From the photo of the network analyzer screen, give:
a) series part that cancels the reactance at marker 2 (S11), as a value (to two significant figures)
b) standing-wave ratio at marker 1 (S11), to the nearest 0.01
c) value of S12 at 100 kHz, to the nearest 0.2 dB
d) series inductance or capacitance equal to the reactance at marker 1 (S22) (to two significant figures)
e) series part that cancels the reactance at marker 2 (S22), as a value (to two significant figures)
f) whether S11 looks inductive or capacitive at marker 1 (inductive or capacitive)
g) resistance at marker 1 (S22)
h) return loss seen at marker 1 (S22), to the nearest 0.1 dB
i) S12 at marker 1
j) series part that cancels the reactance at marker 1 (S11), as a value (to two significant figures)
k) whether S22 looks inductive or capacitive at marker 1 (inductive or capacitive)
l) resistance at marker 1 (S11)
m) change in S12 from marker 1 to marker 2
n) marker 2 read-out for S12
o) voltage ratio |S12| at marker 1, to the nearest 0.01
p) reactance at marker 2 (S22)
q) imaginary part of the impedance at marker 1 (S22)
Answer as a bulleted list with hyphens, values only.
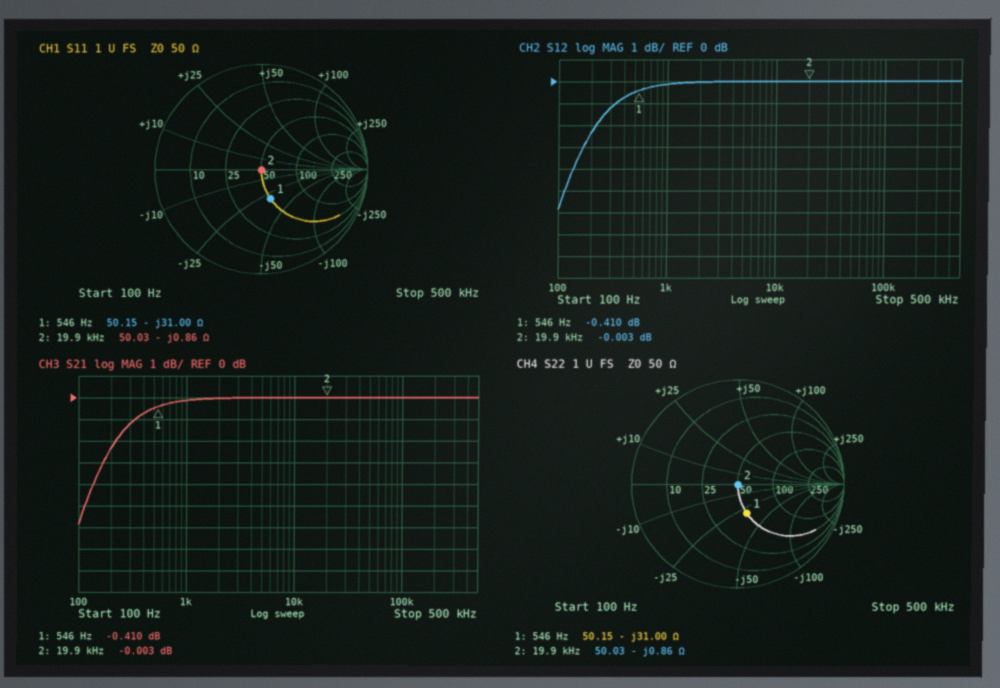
- 6.9 µH
- 1.84
- 0.0 dB
- 9.4 µF
- 6.9 µH
- capacitive
- 50.15 Ω
- 10.6 dB
- -0.410 dB
- 9.0 mH
- capacitive
- 50.15 Ω
- 0.407 dB
- -0.003 dB
- 0.95
- -0.86 Ω
- -31.00 Ω
